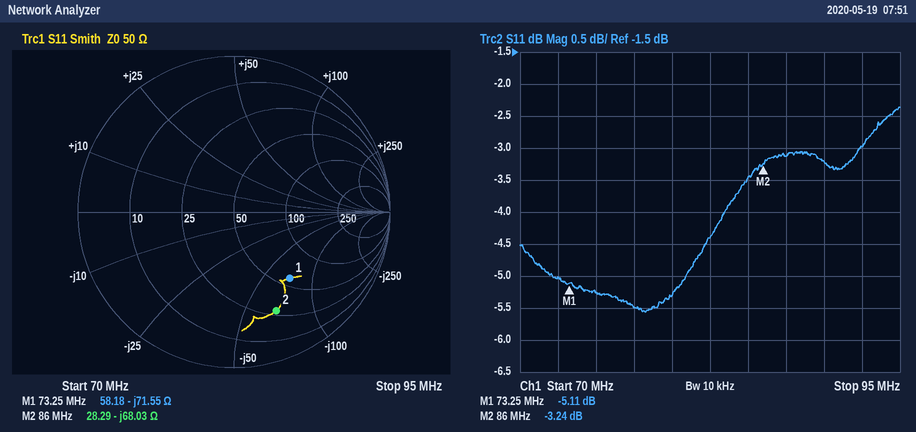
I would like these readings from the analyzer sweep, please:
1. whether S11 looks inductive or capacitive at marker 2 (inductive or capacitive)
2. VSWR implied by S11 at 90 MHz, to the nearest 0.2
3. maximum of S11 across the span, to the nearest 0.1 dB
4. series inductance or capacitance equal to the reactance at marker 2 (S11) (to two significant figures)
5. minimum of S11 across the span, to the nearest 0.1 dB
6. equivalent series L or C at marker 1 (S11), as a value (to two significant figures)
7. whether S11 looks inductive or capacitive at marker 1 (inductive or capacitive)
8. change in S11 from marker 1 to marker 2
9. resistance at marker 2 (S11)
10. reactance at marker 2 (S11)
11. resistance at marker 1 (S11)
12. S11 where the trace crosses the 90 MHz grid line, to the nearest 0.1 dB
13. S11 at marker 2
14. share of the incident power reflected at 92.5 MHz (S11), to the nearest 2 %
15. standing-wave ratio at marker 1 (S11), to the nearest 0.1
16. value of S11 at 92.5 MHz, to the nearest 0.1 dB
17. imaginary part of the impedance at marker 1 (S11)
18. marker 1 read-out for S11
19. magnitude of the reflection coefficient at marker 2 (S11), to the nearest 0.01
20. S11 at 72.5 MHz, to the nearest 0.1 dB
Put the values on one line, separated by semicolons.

capacitive; 5.4; -2.4 dB; 27 pF; -5.6 dB; 30 pF; capacitive; 1.87 dB; 28.29 Ω; -68.03 Ω; 58.18 Ω; -3.2 dB; -3.24 dB; 50 %; 3.5; -3.0 dB; -71.55 Ω; -5.11 dB; 0.69; -5.0 dB
